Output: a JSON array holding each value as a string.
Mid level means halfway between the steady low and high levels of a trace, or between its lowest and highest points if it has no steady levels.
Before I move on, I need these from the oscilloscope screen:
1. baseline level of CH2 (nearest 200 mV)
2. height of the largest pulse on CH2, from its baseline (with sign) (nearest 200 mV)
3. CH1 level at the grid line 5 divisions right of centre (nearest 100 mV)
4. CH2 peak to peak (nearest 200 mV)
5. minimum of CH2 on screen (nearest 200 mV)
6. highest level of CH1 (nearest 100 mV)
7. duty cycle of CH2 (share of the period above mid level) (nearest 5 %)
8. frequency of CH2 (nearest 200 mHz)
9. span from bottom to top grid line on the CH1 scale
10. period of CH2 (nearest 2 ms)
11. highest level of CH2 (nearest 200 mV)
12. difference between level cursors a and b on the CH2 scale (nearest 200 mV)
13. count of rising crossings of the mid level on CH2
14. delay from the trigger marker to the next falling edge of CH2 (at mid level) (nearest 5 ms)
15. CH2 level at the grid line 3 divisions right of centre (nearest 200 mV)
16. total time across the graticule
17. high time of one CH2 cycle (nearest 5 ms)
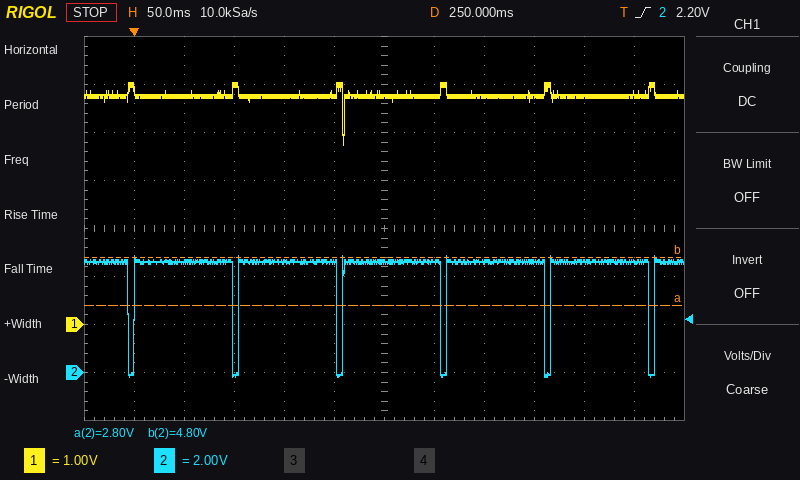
["4.6 V", "-4.8 V", "4.8 V", "5.0 V", "-200 mV", "5.0 V", "95 %", "9.6 Hz", "8 V", "104 ms", "4.8 V", "2.0 V", "6", "100 ms", "4.6 V", "600 ms", "100 ms"]
